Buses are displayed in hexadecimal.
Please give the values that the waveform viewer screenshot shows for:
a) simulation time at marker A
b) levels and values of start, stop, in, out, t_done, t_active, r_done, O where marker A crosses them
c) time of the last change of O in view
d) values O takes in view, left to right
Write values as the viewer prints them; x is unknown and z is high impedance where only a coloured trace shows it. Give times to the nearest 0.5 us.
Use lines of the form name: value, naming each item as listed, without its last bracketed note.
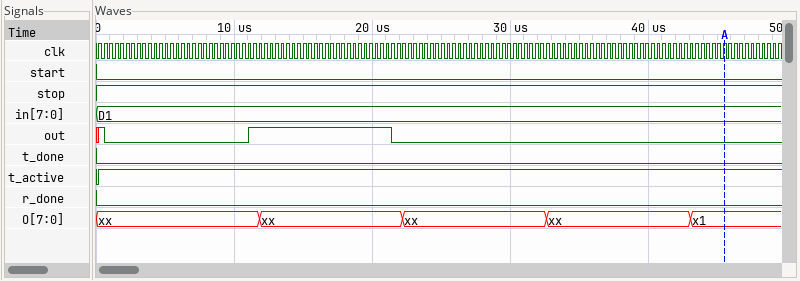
simulation time at marker A: 45.5 us
levels and values of start, stop, in, out, t_done, t_active, r_done, O where marker A crosses them: start=0, stop=1, in=D1, out=0, t_done=0, t_active=1, r_done=0, O=x1
time of the last change of O in view: 43 us
values O takes in view, left to right: xx, xx, xx, xx, x1
